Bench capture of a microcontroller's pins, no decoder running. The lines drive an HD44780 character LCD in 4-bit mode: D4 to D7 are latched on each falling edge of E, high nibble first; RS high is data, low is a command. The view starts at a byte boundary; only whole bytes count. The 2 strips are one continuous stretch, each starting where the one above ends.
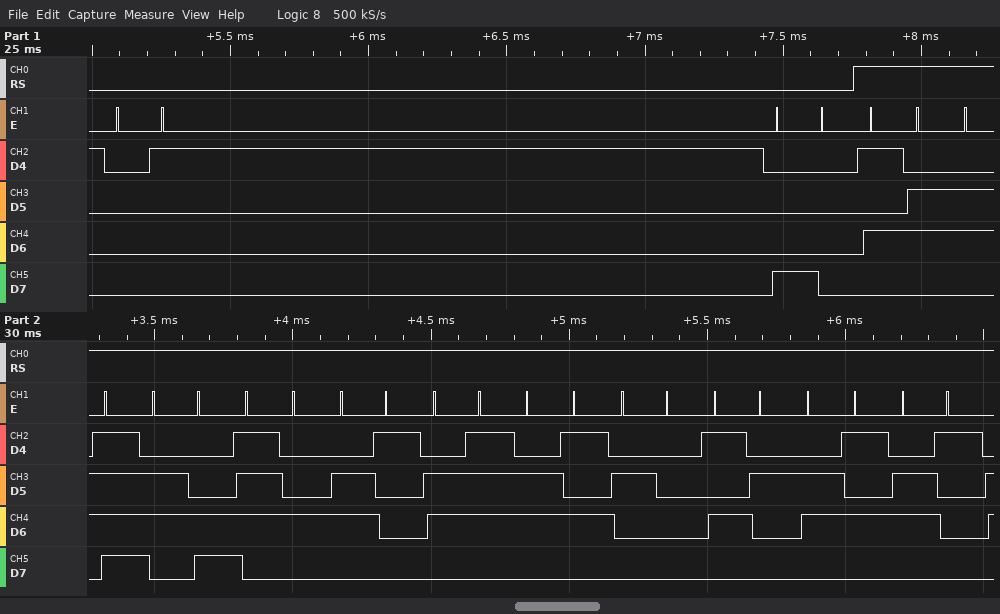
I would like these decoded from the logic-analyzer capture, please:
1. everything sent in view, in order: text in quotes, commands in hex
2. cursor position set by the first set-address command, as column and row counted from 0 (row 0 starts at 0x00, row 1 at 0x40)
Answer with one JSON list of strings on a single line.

["0x01 0x80 \"Voltage Rea\"", "column 0, row 0"]
